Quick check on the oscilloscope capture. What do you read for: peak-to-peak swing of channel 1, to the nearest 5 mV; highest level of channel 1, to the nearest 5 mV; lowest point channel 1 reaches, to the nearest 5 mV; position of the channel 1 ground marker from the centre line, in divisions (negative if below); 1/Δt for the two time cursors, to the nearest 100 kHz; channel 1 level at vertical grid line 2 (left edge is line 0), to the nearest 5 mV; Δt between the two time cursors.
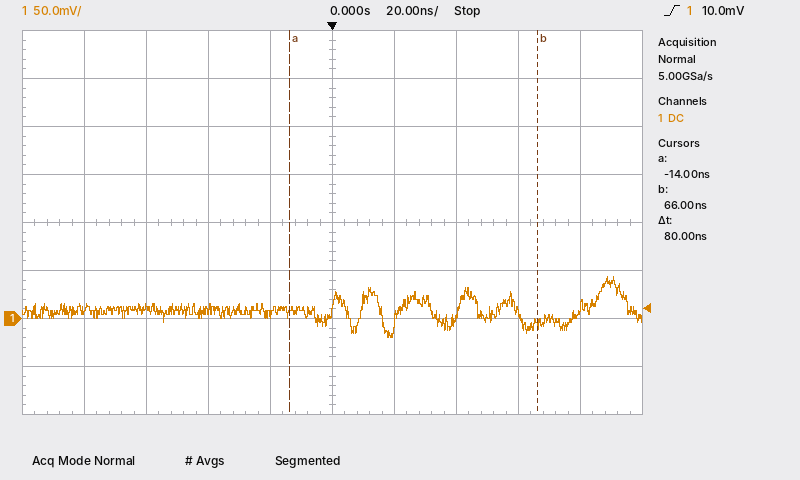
65 mV
45 mV
-20 mV
-2.0 div
12.5 MHz
10 mV
80 ns
